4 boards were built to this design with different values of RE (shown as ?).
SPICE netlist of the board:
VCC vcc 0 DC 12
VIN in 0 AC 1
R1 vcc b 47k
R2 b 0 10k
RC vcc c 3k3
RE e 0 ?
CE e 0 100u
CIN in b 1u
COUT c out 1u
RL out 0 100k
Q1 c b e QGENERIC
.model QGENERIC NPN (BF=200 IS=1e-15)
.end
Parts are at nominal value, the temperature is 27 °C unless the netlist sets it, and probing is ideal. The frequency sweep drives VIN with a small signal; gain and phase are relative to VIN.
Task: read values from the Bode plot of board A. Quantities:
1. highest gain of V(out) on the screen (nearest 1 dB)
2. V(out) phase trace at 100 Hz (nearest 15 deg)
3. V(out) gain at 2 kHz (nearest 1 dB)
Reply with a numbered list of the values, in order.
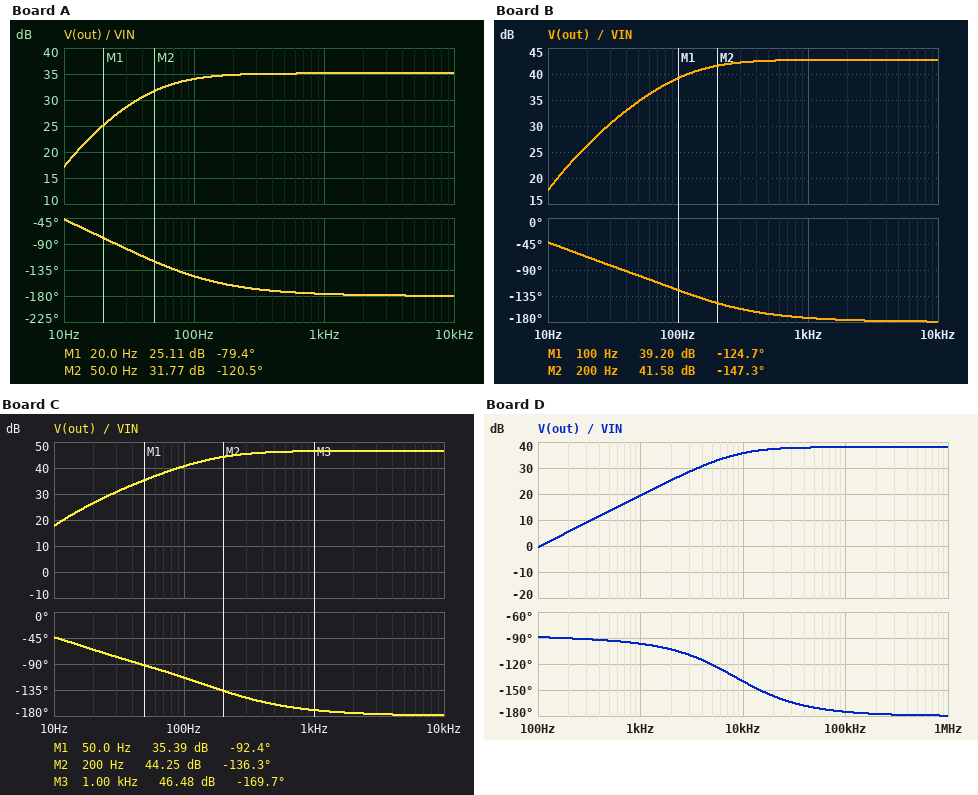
1. 35 dB
2. -150 deg
3. 35 dB
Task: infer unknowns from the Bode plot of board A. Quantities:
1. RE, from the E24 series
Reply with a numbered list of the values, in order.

1. 3 kΩ
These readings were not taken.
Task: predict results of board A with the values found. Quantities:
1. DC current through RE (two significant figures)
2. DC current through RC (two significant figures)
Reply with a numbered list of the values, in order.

1. 460 µA
2. 460 µA
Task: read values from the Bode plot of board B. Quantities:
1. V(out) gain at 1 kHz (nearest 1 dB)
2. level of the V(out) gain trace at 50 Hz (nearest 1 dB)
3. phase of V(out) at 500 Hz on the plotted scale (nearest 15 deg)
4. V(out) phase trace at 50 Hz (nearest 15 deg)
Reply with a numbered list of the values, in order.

1. 43 dB
2. 35 dB
3. -165 deg
4. -105 deg
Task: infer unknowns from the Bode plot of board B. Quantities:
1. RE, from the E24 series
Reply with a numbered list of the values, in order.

1. 1.2 kΩ
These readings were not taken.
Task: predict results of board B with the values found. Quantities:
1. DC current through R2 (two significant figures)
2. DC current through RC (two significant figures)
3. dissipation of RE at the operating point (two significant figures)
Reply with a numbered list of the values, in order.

1. 210 µA
2. 1.1 mA
3. 1.5 mW
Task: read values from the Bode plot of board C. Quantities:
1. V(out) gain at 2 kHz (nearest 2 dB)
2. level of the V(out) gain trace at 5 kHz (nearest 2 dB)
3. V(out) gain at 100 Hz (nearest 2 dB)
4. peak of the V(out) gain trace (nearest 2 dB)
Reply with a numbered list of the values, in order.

1. 46 dB
2. 46 dB
3. 40 dB
4. 46 dB
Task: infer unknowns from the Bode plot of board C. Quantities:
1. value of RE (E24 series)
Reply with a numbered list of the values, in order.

1. 750 Ω
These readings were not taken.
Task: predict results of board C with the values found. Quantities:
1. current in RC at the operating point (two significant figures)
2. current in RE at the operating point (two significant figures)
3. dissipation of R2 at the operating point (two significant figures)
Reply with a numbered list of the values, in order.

1. 1.7 mA
2. 1.7 mA
3. 410 µW
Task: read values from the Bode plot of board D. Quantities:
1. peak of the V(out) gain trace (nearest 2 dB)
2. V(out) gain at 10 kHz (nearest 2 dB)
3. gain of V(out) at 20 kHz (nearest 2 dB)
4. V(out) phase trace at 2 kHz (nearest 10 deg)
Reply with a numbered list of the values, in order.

1. 38 dB
2. 36 dB
3. 38 dB
4. -100 deg
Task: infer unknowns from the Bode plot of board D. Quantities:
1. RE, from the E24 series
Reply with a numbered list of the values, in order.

1. 330 Ω
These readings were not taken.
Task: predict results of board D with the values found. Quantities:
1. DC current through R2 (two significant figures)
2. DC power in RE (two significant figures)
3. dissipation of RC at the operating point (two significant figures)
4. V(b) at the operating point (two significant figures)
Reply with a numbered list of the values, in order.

1. 180 µA
2. 3.6 mW
3. 35 mW
4. 1.8 V
